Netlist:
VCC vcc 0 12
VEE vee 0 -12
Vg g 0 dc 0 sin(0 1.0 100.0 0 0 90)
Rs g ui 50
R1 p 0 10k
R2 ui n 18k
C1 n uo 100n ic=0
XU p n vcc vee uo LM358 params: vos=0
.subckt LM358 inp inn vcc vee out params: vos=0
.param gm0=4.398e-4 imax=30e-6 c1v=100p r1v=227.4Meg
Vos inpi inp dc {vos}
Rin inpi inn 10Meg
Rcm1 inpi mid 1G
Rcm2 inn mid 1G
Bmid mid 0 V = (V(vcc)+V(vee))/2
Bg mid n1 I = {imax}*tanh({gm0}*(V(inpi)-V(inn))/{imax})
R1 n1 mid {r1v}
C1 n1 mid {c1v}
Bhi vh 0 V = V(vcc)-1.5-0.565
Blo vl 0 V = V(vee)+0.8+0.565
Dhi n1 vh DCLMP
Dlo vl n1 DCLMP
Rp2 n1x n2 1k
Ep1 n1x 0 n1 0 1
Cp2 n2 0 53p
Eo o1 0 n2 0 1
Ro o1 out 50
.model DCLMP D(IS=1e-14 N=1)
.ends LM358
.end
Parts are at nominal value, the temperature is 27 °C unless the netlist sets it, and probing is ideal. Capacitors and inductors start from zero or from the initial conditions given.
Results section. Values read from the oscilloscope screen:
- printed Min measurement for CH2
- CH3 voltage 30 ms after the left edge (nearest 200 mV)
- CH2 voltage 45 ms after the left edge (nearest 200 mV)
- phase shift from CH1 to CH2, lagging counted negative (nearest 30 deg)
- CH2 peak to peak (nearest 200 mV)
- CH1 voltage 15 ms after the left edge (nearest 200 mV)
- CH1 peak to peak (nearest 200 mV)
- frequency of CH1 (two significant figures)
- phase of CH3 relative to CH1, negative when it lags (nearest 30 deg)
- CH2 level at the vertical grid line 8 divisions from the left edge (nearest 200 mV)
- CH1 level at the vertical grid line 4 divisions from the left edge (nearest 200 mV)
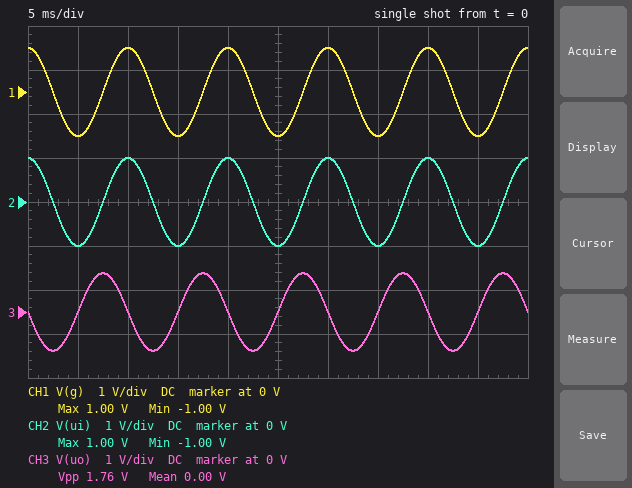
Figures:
-1.00 V
0 V
-1.0 V
0 deg
2.0 V
-1.0 V
2.0 V
100 Hz
90 deg
1.0 V
1.0 V
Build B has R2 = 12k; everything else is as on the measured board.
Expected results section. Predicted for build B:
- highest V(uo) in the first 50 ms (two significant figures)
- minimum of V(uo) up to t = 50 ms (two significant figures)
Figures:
1.3 V
-1.3 V
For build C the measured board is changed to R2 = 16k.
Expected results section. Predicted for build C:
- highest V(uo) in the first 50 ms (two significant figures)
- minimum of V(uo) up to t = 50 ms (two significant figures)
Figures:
990 mV
-990 mV
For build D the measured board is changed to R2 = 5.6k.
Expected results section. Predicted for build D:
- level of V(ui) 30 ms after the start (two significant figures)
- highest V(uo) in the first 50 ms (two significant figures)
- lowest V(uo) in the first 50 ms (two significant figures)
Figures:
990 mV
2.8 V
-2.8 V
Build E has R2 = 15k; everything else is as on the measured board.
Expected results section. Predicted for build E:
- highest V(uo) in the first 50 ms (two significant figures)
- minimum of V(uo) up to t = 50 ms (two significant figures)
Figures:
1.1 V
-1.1 V
